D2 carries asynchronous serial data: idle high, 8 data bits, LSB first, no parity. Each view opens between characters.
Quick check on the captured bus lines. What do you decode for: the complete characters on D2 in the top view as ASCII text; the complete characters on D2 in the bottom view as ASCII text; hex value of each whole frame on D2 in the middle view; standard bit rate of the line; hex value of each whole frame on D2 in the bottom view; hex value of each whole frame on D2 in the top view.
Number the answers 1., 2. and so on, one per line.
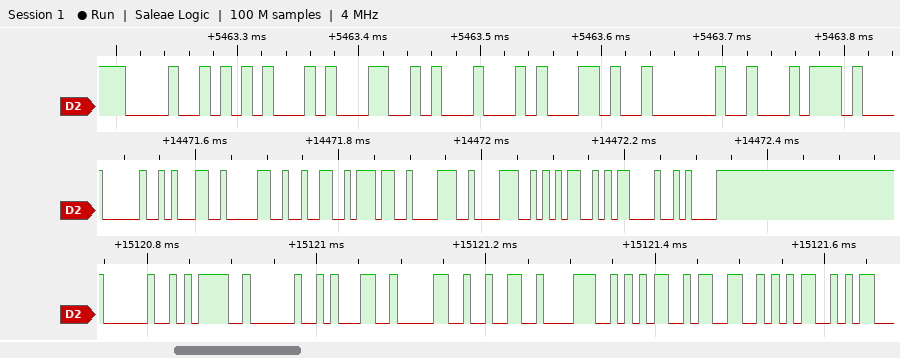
1. "HELD, t"
2. " = 1028535"
3. 20, 31, 30, 32, 37, 38, 38, 35, 0D, 0A
4. 115200 baud
5. 20, 3D, 20, 31, 30, 32, 38, 35, 33, 35
6. 48, 45, 4C, 44, 2C, 20, 74
